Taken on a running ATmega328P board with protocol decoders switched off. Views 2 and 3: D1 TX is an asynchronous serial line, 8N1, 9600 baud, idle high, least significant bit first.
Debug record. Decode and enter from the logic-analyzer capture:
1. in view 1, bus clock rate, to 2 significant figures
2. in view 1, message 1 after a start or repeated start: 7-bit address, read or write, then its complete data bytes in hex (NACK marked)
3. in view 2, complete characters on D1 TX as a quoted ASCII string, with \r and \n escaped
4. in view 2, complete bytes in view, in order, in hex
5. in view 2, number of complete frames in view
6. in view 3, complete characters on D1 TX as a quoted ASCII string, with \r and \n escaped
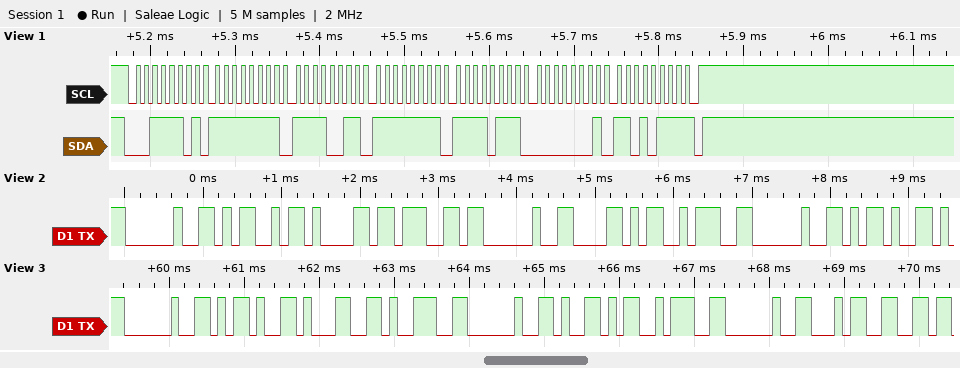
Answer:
100 kHz
0x1E read: FF F3 FF F7 01 D7 NACK
" Mag X: -"
20 4D 61 67 20 58 3A 20 2D
9
" -19 Y: 4"
